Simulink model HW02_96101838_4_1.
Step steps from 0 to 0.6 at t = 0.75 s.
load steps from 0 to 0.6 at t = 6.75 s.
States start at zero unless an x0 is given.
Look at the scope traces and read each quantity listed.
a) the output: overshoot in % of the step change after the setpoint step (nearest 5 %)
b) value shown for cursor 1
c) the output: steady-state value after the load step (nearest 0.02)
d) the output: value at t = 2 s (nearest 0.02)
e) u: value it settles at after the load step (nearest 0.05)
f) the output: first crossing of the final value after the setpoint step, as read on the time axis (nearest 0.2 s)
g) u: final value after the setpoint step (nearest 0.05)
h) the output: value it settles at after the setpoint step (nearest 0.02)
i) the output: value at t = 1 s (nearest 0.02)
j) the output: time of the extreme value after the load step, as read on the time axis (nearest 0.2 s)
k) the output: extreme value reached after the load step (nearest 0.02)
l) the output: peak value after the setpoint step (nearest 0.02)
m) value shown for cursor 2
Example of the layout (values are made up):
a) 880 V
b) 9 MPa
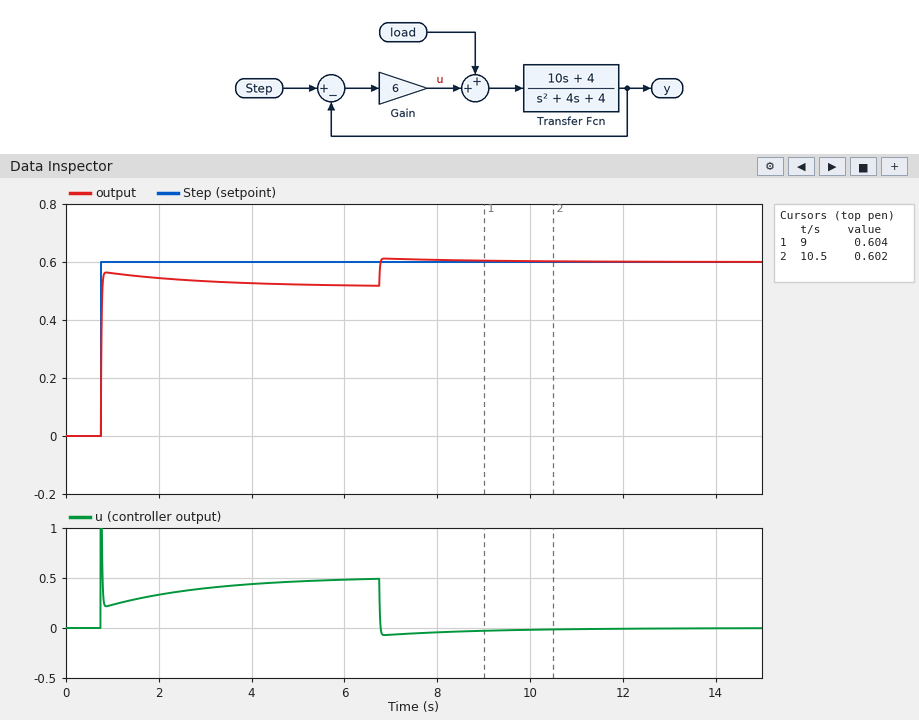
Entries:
a) 10 %
b) 0.604
c) 0.60
d) 0.54
e) 0.00
f) 0.8 s
g) 0.50
h) 0.52
i) 0.56
j) 6.8 s
k) 0.62
l) 0.56
m) 0.602
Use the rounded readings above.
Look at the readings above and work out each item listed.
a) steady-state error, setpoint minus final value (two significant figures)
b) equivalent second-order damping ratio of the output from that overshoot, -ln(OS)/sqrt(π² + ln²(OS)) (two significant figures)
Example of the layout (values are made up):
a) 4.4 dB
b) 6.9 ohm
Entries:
a) 0.080
b) 0.59
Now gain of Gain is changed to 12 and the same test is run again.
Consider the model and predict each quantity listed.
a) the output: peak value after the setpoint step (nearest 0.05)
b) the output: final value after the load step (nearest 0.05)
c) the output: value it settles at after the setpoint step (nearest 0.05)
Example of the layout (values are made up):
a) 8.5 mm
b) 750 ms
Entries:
a) 0.60
b) 0.60
c) 0.55
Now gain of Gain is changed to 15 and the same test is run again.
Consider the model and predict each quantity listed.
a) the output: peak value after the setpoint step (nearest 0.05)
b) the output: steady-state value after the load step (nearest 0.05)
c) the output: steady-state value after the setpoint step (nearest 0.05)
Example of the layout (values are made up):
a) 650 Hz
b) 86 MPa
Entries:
a) 0.60
b) 0.60
c) 0.55
